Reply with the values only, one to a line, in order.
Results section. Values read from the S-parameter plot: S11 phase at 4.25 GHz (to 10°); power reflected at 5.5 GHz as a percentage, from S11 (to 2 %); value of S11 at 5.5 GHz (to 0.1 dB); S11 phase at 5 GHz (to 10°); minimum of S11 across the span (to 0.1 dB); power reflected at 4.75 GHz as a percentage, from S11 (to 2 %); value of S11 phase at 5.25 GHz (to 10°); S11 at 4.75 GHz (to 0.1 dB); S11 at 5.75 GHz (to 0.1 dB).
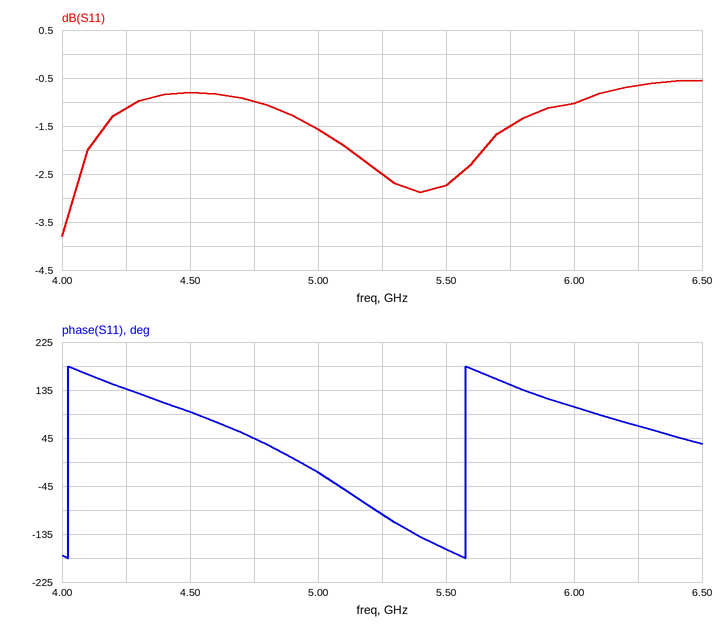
140°
54 %
-2.7 dB
-20°
-3.8 dB
80 %
-100°
-1.0 dB
-1.5 dB
